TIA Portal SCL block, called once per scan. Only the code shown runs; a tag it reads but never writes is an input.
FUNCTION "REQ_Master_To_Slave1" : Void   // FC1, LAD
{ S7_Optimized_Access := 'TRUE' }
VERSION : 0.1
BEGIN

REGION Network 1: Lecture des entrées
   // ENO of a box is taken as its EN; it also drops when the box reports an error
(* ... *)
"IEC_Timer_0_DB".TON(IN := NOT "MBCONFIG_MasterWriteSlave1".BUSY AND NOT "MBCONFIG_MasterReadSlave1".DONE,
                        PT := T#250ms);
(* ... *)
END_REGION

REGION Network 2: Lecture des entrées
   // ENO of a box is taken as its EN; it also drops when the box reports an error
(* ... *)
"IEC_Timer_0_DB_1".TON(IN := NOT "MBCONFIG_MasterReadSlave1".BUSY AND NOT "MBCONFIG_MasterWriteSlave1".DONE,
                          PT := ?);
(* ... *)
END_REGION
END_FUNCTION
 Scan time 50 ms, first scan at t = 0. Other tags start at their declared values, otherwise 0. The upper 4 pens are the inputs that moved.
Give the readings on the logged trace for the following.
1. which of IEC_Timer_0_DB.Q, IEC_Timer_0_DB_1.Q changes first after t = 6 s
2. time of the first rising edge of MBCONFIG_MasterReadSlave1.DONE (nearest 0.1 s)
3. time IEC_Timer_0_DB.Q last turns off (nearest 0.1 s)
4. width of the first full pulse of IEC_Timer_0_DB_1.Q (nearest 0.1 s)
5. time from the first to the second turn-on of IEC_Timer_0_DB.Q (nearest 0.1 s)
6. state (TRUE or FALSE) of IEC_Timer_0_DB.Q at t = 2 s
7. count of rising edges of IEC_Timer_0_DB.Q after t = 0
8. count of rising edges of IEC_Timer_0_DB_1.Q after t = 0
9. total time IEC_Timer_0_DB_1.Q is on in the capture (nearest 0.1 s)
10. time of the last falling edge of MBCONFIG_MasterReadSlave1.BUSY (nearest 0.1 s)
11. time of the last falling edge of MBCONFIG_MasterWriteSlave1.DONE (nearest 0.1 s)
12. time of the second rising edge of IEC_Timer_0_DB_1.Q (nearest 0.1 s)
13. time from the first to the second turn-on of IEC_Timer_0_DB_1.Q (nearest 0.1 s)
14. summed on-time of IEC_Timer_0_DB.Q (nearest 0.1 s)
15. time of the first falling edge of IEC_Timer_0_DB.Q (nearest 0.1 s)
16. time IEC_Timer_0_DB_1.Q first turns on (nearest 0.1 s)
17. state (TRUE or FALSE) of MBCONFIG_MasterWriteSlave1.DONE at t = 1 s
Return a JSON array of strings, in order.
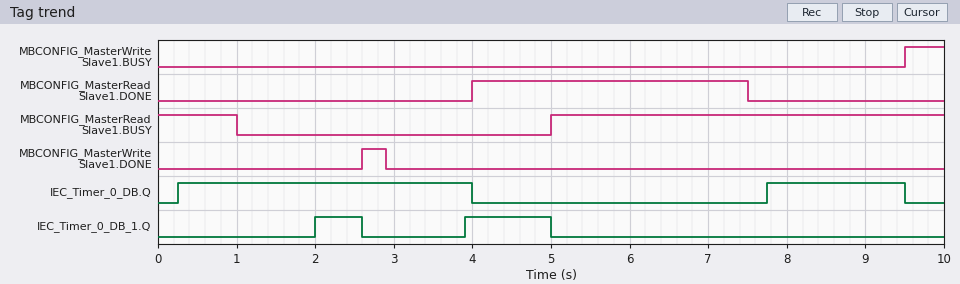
["IEC_Timer_0_DB.Q", "4.0 s", "9.5 s", "0.6 s", "7.5 s", "TRUE", "2", "2", "1.7 s", "1.0 s", "2.9 s", "3.9 s", "1.9 s", "5.5 s", "4.0 s", "2.0 s", "FALSE"]
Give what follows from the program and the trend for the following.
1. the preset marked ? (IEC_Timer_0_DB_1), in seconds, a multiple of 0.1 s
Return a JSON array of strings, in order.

["1.0 s"]
